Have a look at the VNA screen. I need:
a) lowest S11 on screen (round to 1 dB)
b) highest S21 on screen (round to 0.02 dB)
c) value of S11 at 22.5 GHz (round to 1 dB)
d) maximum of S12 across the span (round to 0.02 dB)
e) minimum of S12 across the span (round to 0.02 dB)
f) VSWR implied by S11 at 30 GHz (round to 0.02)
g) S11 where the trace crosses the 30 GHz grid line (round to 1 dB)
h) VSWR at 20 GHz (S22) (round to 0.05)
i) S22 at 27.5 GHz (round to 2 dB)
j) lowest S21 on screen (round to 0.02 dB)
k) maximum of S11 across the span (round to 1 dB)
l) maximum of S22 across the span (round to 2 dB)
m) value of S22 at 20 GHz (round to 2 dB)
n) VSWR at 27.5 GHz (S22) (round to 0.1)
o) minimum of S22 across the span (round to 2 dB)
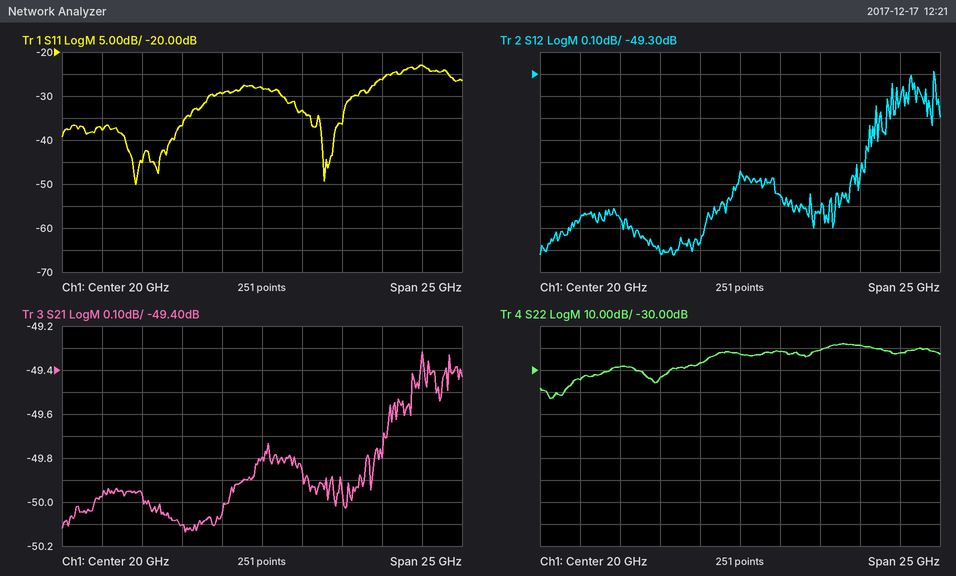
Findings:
-50 dB
-49.32 dB
-33 dB
-49.28 dB
-50.12 dB
1.16
-23 dB
1.15
-18 dB
-50.14 dB
-23 dB
-18 dB
-22 dB
1.3
-42 dB
